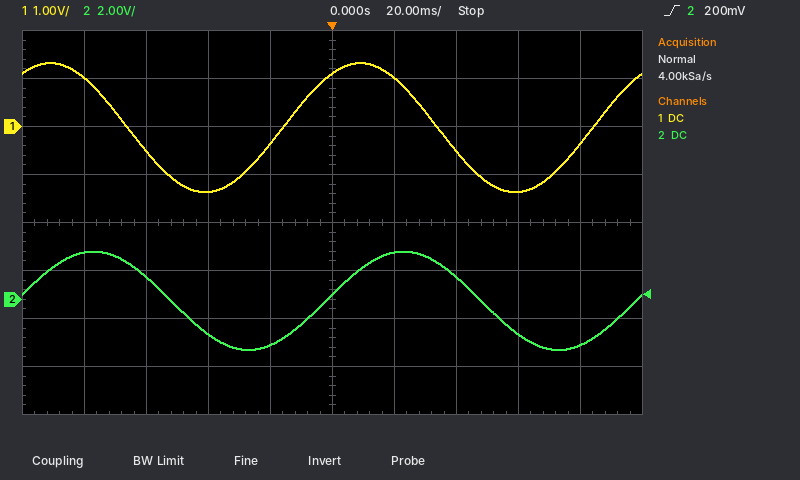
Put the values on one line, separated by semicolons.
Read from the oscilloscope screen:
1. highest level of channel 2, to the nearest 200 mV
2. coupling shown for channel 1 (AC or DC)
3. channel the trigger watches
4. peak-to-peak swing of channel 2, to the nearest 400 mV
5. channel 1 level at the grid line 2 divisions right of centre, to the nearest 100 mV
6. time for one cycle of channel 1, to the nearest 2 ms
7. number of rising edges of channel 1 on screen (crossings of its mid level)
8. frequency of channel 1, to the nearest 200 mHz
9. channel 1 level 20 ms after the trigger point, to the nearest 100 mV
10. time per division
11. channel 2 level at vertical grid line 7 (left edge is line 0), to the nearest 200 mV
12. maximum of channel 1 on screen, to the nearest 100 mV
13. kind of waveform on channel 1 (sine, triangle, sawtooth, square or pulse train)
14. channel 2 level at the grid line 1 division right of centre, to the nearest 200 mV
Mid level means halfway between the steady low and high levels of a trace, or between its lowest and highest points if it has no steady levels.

2.0 V; DC; channel 2; 4.0 V; -500 mV; 100 ms; 2; 10.0 Hz; 1.0 V; 20 ms; 1.0 V; 1.3 V; sine; 2.0 V
